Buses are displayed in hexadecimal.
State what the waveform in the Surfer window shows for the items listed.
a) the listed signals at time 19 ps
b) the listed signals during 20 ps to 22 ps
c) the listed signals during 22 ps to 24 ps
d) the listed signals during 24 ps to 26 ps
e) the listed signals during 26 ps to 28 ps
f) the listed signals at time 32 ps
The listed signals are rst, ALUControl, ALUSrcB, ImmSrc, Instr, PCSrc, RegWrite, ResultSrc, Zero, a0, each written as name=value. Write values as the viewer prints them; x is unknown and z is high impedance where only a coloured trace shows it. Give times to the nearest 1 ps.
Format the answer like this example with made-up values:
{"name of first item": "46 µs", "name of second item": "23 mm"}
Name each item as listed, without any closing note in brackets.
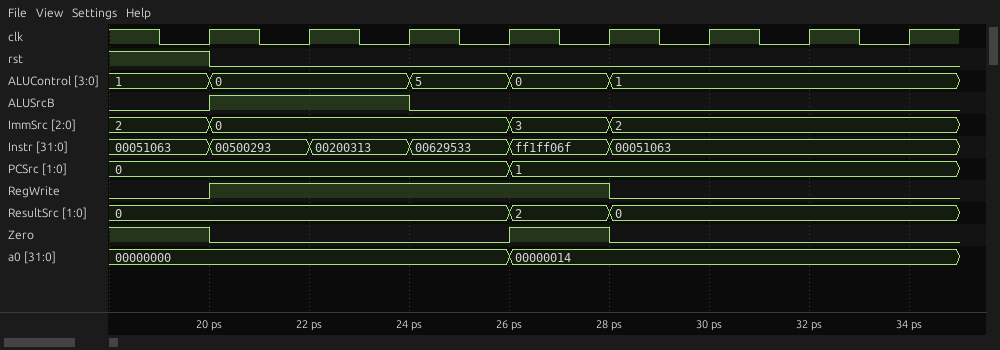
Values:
{"the listed signals at time 19 ps": "rst=1, ALUControl=1, ALUSrcB=0, ImmSrc=2, Instr=00051063, PCSrc=0, RegWrite=0, ResultSrc=0, Zero=1, a0=00000000", "the listed signals during 20 ps to 22 ps": "rst=0, ALUControl=0, ALUSrcB=1, ImmSrc=0, Instr=00500293, PCSrc=0, RegWrite=1, ResultSrc=0, Zero=0, a0=00000000", "the listed signals during 22 ps to 24 ps": "rst=0, ALUControl=0, ALUSrcB=1, ImmSrc=0, Instr=00200313, PCSrc=0, RegWrite=1, ResultSrc=0, Zero=0, a0=00000000", "the listed signals during 24 ps to 26 ps": "rst=0, ALUControl=5, ALUSrcB=0, ImmSrc=0, Instr=00629533, PCSrc=0, RegWrite=1, ResultSrc=0, Zero=0, a0=00000000", "the listed signals during 26 ps to 28 ps": "rst=0, ALUControl=0, ALUSrcB=0, ImmSrc=3, Instr=ff1ff06f, PCSrc=1, RegWrite=1, ResultSrc=2, Zero=1, a0=00000014", "the listed signals at time 32 ps": "rst=0, ALUControl=1, ALUSrcB=0, ImmSrc=2, Instr=00051063, PCSrc=1, RegWrite=0, ResultSrc=0, Zero=0, a0=00000014"}
